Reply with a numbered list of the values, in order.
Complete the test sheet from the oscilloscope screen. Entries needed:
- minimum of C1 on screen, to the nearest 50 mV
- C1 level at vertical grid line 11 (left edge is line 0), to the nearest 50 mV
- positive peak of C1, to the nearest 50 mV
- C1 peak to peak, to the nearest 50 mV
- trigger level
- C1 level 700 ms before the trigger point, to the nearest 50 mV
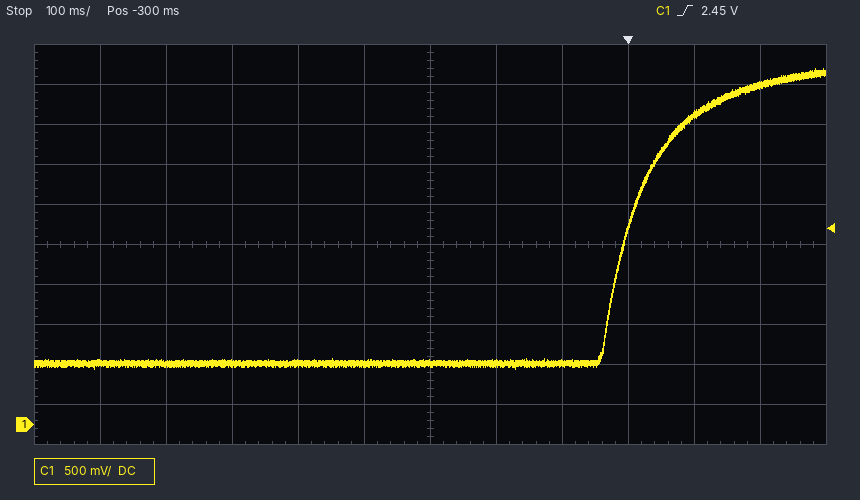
1. 700 mV
2. 4.25 V
3. 4.45 V
4. 3.75 V
5. 2.45 V
6. 750 mV
